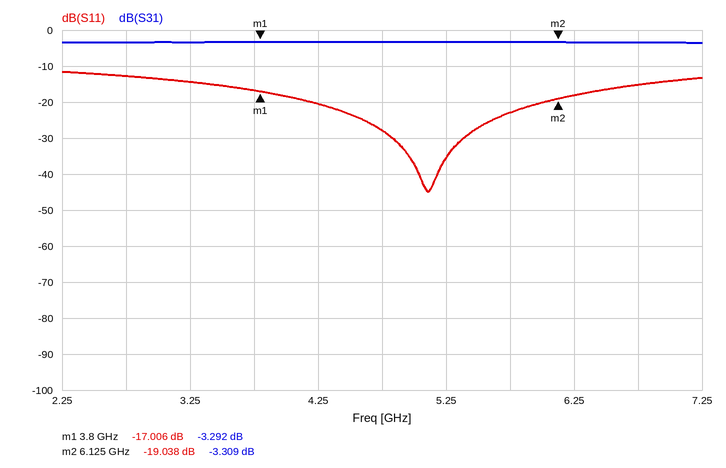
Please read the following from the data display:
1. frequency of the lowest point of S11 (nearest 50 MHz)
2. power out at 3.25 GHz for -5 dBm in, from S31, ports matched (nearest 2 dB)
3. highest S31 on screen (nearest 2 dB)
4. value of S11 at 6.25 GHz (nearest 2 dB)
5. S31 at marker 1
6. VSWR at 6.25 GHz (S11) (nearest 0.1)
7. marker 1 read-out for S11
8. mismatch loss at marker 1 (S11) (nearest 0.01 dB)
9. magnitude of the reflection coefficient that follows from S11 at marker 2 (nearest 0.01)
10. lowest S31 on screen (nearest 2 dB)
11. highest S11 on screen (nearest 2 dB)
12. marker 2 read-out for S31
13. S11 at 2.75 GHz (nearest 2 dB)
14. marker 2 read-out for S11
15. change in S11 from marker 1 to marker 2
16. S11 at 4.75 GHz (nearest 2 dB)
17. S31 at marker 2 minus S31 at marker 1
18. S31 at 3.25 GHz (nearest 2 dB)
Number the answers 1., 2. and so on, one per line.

1. 5.10 GHz
2. -8 dBm
3. -4 dB
4. -18 dB
5. -3.292 dB
6. 1.3
7. -17.006 dB
8. 0.09 dB
9. 0.11
10. -4 dB
11. -12 dB
12. -3.309 dB
13. -12 dB
14. -19.038 dB
15. -2.032 dB
16. -28 dB
17. -0.017 dB
18. -4 dB
